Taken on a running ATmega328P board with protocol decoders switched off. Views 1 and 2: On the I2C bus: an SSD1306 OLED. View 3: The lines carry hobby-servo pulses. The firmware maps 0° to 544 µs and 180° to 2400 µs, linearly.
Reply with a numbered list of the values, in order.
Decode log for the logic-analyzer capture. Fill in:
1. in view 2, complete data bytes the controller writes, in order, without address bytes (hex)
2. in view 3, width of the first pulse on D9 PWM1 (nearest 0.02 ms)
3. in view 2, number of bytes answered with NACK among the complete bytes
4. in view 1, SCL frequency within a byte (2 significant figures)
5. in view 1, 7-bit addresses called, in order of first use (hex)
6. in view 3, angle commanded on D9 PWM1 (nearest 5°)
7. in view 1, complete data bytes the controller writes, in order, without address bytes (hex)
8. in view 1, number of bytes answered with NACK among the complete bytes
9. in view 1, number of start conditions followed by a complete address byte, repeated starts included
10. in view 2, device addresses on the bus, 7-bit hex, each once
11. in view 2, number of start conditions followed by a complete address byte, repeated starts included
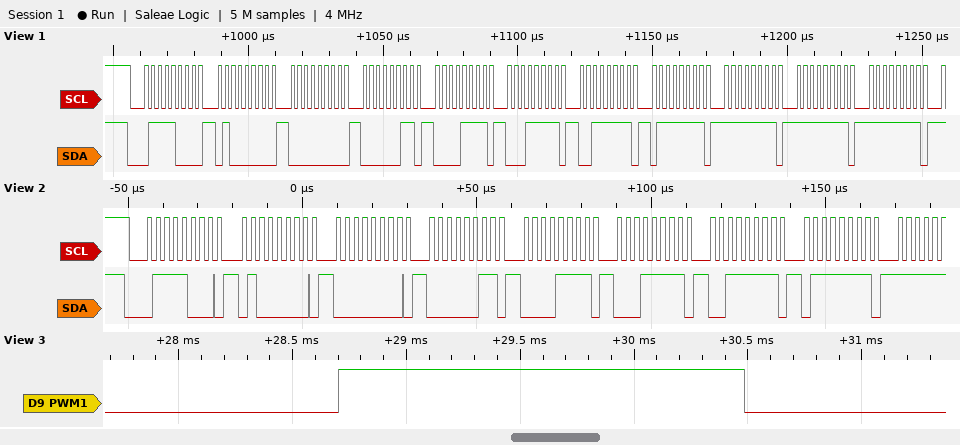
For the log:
1. 40 00 03 0F 1F 3F 7F
2. 1.78 ms
3. 0
4. 400 kHz
5. 0x3C
6. 120°
7. 40 00 03 0F 1F 3F 7F FF FF FF
8. 0
9. 1
10. 0x3C
11. 1
